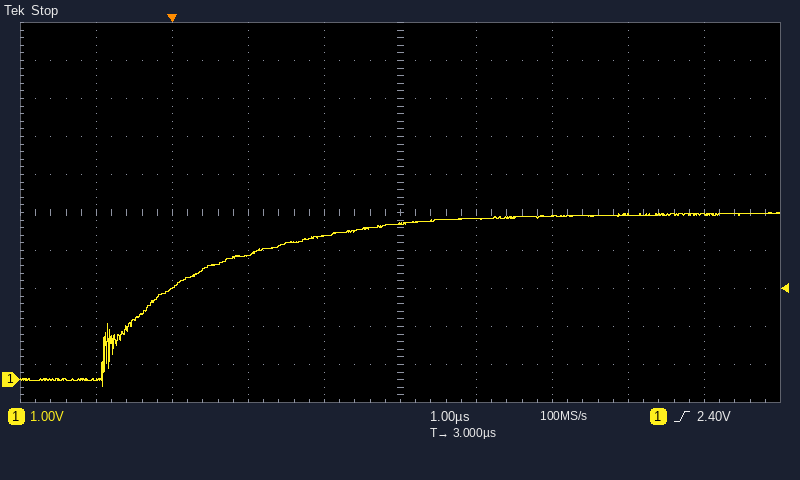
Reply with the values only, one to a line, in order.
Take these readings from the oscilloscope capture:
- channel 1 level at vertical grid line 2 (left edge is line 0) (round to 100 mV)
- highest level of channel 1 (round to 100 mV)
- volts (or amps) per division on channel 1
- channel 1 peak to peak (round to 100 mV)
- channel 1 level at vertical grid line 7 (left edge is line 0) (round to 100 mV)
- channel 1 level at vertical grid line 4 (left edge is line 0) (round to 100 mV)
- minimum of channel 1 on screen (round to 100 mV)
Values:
2.4 V
4.4 V
1 V
4.6 V
4.3 V
3.8 V
-200 mV
